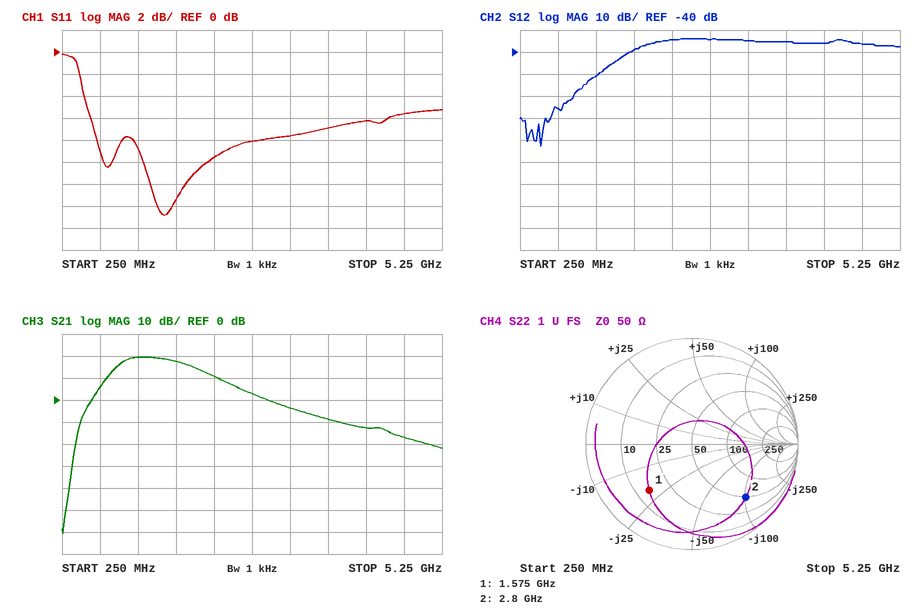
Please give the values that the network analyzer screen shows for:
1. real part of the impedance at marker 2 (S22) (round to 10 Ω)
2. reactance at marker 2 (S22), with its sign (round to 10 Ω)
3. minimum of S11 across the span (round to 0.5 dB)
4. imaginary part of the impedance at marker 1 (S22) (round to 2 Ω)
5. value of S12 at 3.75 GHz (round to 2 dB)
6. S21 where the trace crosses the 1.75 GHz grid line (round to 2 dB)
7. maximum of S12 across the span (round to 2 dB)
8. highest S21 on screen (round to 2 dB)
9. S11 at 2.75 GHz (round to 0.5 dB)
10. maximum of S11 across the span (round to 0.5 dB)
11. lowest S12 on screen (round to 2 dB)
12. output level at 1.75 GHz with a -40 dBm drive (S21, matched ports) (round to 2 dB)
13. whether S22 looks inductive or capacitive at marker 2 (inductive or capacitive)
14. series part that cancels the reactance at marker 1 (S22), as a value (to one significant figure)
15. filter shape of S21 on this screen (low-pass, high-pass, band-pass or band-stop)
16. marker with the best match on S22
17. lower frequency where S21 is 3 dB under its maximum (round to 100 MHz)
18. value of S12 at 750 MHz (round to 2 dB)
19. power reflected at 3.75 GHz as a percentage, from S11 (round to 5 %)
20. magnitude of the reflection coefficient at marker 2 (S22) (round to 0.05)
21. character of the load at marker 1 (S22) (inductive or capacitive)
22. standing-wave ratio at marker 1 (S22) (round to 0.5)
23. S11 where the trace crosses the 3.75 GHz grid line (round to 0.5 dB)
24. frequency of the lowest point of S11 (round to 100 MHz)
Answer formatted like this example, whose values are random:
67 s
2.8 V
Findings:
50 Ω
-100 Ω
-15.0 dB
-20 Ω
-36 dB
18 dB
-34 dB
20 dB
-8.0 dB
0.0 dB
-82 dB
-22 dBm
capacitive
2 nH
band-pass
marker 1
1.0 GHz
-66 dB
20 %
0.70
capacitive
4.0
-7.0 dB
1.6 GHz
